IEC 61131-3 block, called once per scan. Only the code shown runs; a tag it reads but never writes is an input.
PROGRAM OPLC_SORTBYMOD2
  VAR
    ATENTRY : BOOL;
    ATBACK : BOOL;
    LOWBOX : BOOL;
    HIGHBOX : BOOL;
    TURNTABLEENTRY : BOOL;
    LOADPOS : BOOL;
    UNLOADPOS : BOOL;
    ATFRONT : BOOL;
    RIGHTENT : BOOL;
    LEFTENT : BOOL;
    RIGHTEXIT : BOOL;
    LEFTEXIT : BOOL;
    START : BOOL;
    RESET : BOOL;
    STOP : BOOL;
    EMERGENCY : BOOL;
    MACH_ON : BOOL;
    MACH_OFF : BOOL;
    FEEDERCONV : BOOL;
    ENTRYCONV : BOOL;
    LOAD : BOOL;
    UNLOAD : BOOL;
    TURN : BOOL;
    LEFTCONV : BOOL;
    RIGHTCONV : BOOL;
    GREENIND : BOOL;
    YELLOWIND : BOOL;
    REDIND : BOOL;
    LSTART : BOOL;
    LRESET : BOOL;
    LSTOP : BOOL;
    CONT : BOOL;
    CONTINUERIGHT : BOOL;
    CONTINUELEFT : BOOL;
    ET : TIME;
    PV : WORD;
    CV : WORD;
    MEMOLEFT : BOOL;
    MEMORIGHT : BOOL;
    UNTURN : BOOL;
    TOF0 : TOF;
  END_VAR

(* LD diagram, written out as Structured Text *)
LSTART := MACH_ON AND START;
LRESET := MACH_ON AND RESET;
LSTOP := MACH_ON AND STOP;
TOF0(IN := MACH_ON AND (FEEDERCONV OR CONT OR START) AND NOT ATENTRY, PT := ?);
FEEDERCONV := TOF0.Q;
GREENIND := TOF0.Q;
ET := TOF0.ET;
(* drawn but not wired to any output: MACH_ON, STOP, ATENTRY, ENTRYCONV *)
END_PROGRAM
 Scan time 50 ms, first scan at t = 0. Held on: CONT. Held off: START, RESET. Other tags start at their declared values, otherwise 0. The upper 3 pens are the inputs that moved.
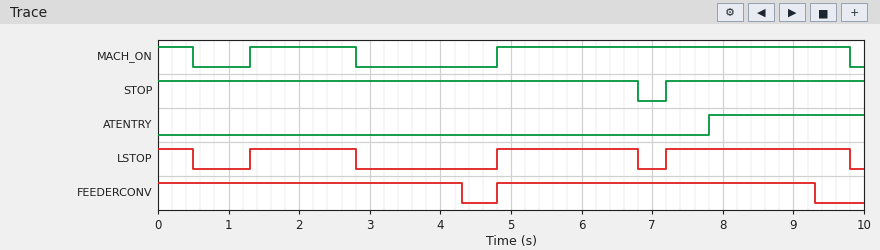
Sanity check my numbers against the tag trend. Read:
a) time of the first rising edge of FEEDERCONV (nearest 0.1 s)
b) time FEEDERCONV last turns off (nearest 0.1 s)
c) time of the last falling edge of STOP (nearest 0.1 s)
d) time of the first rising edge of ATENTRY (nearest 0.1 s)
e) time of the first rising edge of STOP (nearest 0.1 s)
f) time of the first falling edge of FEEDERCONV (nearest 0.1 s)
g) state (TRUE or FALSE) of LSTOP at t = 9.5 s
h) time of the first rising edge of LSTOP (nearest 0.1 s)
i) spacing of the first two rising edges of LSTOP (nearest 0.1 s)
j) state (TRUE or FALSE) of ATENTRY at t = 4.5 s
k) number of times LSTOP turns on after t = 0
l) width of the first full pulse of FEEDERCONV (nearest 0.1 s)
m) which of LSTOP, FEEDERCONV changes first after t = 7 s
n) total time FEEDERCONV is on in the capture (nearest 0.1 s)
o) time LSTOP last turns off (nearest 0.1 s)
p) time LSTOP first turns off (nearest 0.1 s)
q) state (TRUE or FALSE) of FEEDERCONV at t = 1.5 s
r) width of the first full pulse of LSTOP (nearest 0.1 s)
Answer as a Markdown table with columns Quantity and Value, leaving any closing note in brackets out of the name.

| Quantity | Value |
|---|---|
| time of the first rising edge of FEEDERCONV | 4.8 s |
| time FEEDERCONV last turns off | 9.3 s |
| time of the last falling edge of STOP | 6.8 s |
| time of the first rising edge of ATENTRY | 7.8 s |
| time of the first rising edge of STOP | 7.2 s |
| time of the first falling edge of FEEDERCONV | 4.3 s |
| state (TRUE or FALSE) of LSTOP at t = 9.5 s | TRUE |
| time of the first rising edge of LSTOP | 1.3 s |
| spacing of the first two rising edges of LSTOP | 3.5 s |
| state (TRUE or FALSE) of ATENTRY at t = 4.5 s | FALSE |
| number of times LSTOP turns on after t = 0 | 3 |
| width of the first full pulse of FEEDERCONV | 4.5 s |
| which of LSTOP, FEEDERCONV changes first after t = 7 s | LSTOP |
| total time FEEDERCONV is on in the capture | 8.8 s |
| time LSTOP last turns off | 9.8 s |
| time LSTOP first turns off | 0.5 s |
| state (TRUE or FALSE) of FEEDERCONV at t = 1.5 s | TRUE |
| width of the first full pulse of LSTOP | 1.5 s |
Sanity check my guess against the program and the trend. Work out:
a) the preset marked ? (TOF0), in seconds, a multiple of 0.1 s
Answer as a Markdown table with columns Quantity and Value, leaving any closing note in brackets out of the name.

| Quantity | Value |
|---|---|
| the preset marked ? (TOF0), in seconds, a multiple of 0.1 s | 1.5 s |
